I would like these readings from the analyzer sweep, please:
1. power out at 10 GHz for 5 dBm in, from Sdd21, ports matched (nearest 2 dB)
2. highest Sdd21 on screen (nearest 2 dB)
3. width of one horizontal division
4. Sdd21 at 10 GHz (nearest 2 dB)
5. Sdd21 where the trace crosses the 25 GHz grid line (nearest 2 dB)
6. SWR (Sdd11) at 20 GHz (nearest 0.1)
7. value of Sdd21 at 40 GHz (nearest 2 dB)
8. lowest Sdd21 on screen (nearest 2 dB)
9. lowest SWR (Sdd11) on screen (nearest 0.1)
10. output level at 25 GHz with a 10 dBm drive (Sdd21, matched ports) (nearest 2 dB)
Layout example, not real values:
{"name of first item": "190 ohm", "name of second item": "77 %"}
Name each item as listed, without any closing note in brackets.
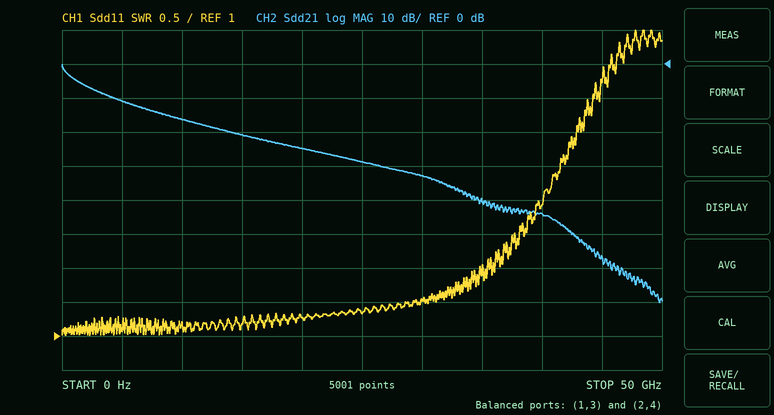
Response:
{"power out at 10 GHz for 5 dBm in, from Sdd21, ports matched": "-12 dBm", "highest Sdd21 on screen": "0 dB", "width of one horizontal division": "5 GHz", "Sdd21 at 10 GHz": "-16 dB", "Sdd21 where the trace crosses the 25 GHz grid line": "-28 dB", "SWR (Sdd11) at 20 GHz": "1.3", "value of Sdd21 at 40 GHz": "-44 dB", "lowest Sdd21 on screen": "-70 dB", "lowest SWR (Sdd11) on screen": "1.0", "output level at 25 GHz with a 10 dBm drive (Sdd21, matched ports)": "-18 dBm"}
